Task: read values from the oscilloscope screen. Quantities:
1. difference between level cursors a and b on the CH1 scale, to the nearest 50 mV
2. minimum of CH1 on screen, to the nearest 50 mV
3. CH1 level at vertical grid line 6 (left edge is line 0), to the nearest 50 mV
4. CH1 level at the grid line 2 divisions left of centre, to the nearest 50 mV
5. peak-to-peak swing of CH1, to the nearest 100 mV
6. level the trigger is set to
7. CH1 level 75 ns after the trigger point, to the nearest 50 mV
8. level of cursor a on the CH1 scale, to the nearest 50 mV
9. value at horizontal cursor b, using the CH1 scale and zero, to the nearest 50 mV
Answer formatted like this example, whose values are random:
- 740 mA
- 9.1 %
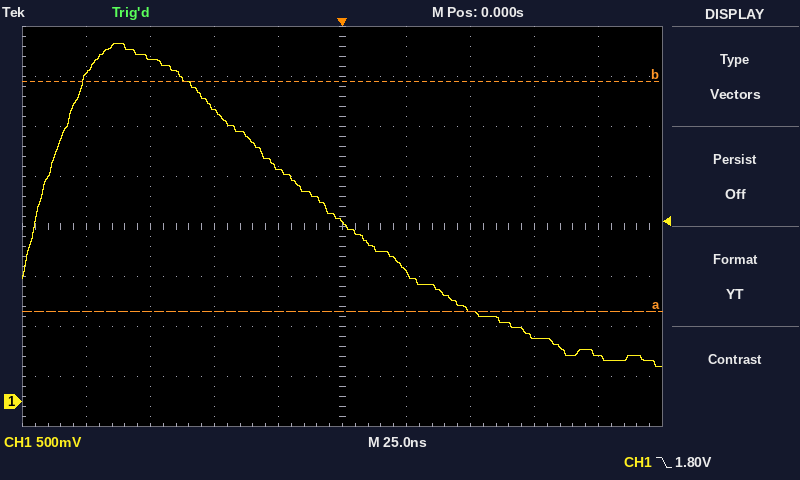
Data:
- 2.30 V
- 350 mV
- 1.30 V
- 2.90 V
- 3.20 V
- 1.80 V
- 650 mV
- 900 mV
- 3.20 V
